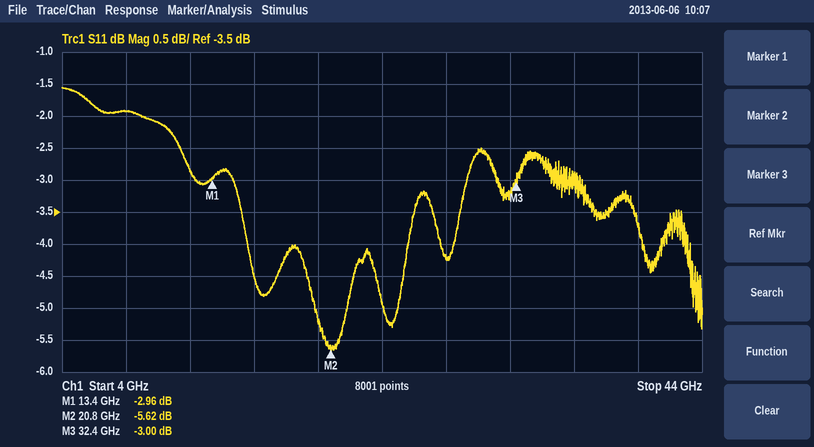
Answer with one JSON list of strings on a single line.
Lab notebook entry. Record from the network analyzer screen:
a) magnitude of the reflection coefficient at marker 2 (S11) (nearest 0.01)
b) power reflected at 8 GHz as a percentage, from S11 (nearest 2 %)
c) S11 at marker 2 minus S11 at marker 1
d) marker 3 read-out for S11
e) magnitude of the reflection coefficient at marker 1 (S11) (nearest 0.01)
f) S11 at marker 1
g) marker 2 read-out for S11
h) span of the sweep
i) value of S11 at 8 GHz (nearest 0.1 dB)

["0.52", "64 %", "-2.66 dB", "-3.00 dB", "0.71", "-2.96 dB", "-5.62 dB", "40 GHz", "-1.9 dB"]
